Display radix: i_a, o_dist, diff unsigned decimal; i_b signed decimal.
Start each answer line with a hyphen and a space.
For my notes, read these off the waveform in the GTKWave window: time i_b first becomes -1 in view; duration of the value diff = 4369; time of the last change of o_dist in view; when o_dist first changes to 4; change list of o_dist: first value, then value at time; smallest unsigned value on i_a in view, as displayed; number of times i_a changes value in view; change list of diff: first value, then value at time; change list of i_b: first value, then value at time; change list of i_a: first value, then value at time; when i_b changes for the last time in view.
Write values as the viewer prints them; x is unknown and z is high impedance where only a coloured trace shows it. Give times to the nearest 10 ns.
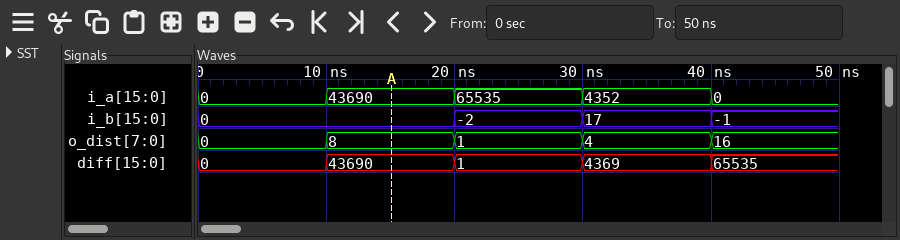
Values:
- 40 ns
- 10 ns
- 40 ns
- 30 ns
- 0, 8 at 10 ns, 1 at 20 ns, 4 at 30 ns, 16 at 40 ns
- 0
- 4
- 0, 43690 at 10 ns, 1 at 20 ns, 4369 at 30 ns, 65535 at 40 ns
- 0, -2 at 20 ns, 17 at 30 ns, -1 at 40 ns
- 0, 43690 at 10 ns, 65535 at 20 ns, 4352 at 30 ns, 0 at 40 ns
- 40 ns
